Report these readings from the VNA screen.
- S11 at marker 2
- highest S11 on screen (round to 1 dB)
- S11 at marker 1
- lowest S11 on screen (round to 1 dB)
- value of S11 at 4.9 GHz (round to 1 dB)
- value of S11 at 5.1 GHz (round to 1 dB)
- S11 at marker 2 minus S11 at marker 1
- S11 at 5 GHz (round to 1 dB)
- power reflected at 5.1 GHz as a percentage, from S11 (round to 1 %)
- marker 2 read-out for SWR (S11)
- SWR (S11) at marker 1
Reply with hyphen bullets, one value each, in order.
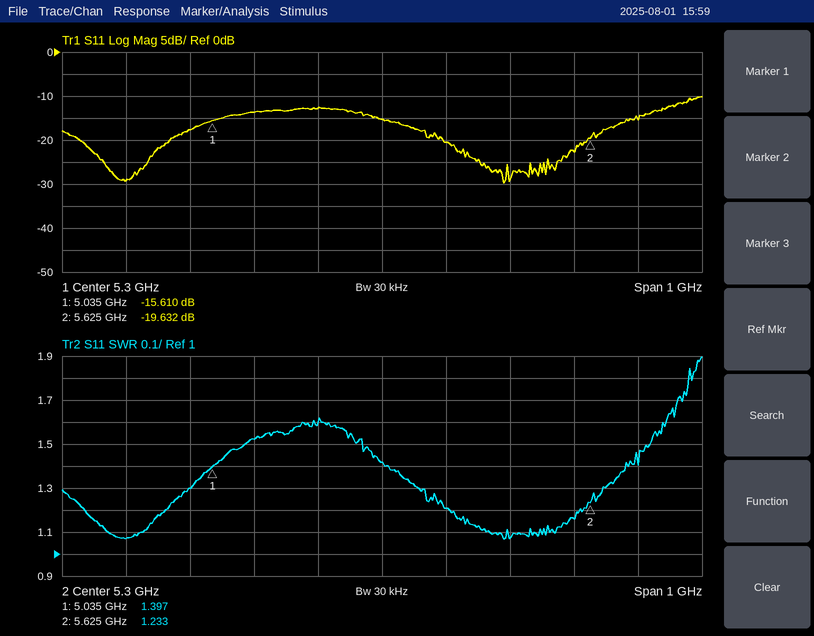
- -19.632 dB
- -10 dB
- -15.610 dB
- -30 dB
- -29 dB
- -14 dB
- -4.022 dB
- -18 dB
- 4 %
- 1.233
- 1.397
